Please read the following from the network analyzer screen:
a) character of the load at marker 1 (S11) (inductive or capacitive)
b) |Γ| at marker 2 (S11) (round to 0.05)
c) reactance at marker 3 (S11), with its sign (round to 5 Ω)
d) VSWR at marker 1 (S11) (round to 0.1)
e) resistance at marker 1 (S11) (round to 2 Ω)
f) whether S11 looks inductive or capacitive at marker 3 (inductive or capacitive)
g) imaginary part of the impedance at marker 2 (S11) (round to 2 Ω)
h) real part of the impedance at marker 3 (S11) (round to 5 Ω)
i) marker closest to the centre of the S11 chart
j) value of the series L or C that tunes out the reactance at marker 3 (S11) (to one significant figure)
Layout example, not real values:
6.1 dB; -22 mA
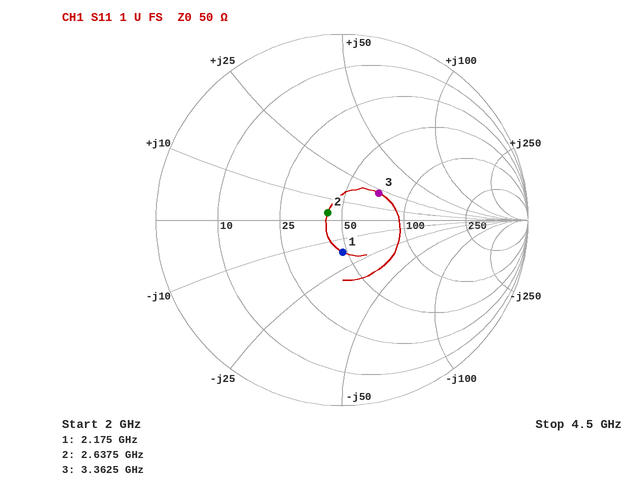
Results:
capacitive; 0.10; +20 Ω; 1.4; 48 Ω; inductive; +4 Ω; 70 Ω; marker 2; 2 pF
